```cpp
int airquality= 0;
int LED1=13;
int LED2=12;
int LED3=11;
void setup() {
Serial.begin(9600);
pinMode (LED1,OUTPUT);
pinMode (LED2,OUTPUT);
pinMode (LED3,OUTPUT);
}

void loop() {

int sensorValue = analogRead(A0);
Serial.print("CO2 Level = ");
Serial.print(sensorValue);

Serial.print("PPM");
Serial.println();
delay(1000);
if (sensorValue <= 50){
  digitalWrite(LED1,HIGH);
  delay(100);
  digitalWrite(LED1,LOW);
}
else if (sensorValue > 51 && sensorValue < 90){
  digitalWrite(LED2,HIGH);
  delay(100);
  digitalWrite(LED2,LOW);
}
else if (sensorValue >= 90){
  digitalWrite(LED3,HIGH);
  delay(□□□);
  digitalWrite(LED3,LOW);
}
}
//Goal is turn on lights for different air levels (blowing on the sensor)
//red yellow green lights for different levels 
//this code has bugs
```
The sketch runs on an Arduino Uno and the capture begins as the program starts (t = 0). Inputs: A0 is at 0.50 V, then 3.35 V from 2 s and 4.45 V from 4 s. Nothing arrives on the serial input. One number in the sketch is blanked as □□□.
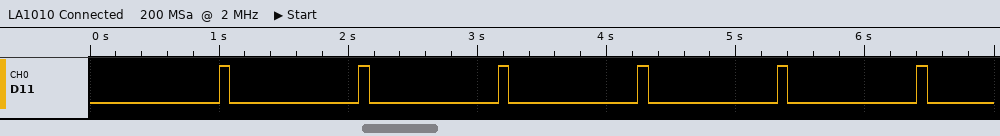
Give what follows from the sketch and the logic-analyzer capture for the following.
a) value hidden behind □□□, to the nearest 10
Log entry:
80
